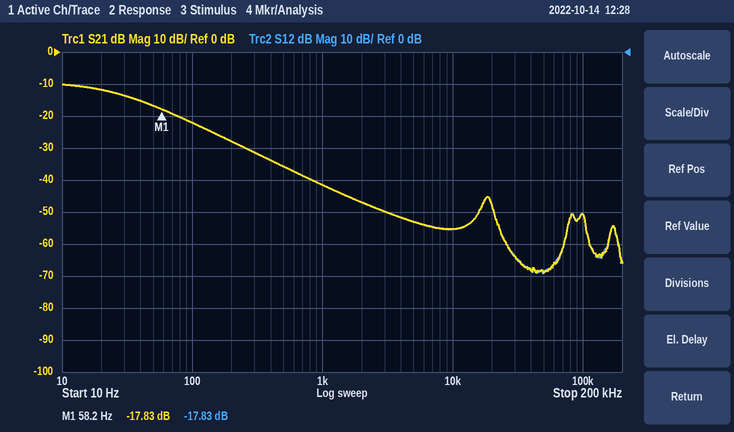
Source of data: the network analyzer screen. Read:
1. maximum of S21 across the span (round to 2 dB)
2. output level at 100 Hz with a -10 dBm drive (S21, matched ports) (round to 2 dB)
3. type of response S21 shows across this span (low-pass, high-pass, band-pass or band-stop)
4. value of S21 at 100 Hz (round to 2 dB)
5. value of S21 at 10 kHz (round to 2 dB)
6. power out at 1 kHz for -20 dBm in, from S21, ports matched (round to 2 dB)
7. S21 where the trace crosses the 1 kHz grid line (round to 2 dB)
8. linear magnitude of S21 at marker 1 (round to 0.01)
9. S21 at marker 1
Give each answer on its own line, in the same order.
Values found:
-10 dB
-32 dBm
low-pass
-22 dB
-56 dB
-62 dBm
-42 dB
0.13
-17.83 dB
